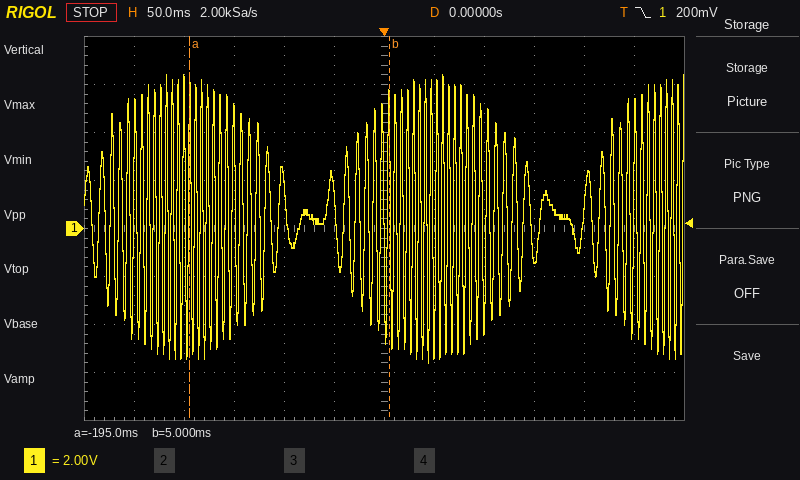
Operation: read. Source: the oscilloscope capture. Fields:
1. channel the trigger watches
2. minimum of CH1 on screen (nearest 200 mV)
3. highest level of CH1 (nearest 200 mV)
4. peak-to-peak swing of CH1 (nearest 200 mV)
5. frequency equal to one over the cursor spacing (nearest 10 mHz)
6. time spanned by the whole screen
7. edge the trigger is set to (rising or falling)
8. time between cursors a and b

CH1
-5.6 V
6.4 V
12.0 V
5.00 Hz
600 ms
falling
200 ms
